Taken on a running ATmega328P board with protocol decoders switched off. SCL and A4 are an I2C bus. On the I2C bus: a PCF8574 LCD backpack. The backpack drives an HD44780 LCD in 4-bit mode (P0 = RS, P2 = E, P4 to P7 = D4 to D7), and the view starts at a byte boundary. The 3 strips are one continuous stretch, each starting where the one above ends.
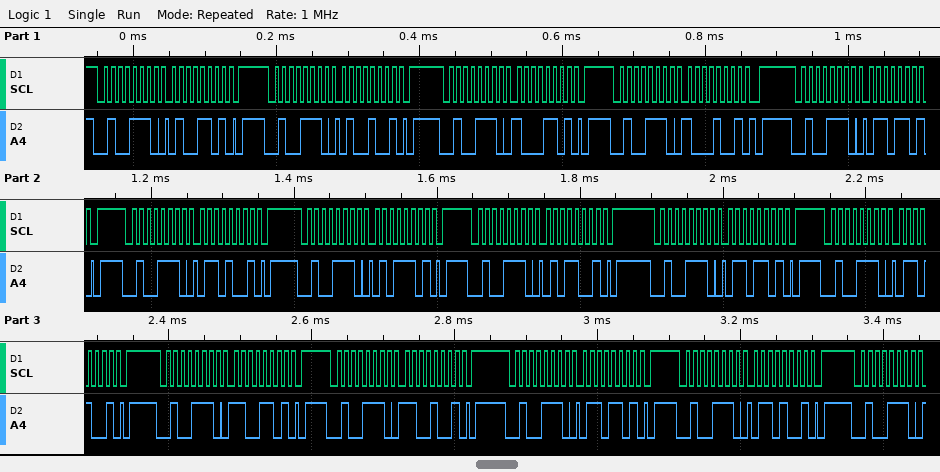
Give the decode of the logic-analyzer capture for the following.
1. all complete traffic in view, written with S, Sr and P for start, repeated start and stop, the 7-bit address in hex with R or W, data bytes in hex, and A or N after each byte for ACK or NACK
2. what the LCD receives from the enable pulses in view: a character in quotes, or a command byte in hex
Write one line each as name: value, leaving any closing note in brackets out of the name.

all complete traffic in view, written with S, Sr and P for start, repeated start and stop, the 7-bit address in hex with R or W, data bytes in hex, and A or N after each byte for ACK or NACK: S 27W A 4D A P S 27W A 49 A P S 27W A 8D A P S 27W A 89 A P S 27W A 6D A P S 27W A 69 A P S 27W A 5D A P S 27W A 59 A P S 27W A 6D A P S 27W A 69 A P S 27W A CD A P S 27W A C9 A P S 27W A 6D A P S 27W A 69 A P S 27W A
what the LCD receives from the enable pulses in view: a character in quotes, or a command byte in hex: 'H' 'e' 'l'
